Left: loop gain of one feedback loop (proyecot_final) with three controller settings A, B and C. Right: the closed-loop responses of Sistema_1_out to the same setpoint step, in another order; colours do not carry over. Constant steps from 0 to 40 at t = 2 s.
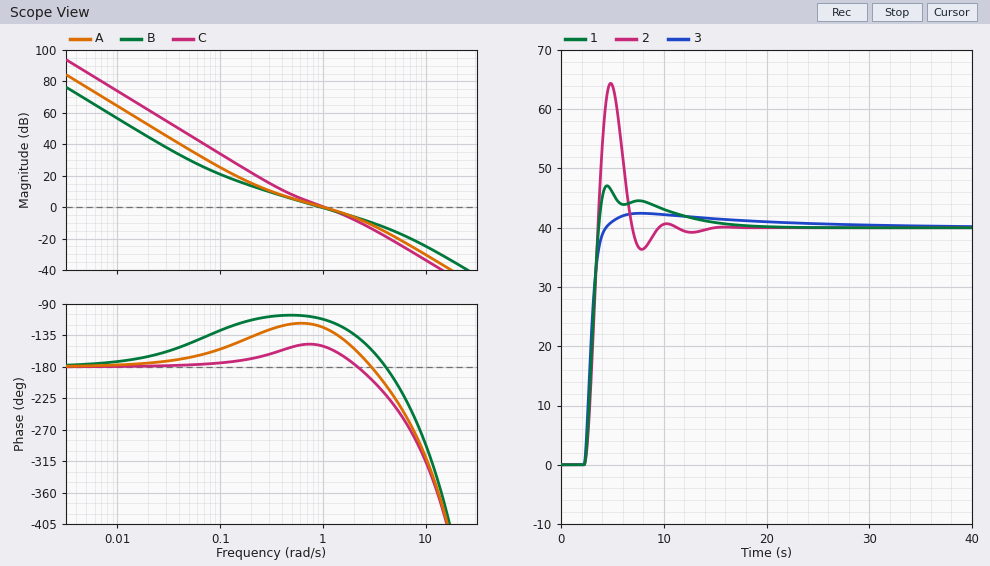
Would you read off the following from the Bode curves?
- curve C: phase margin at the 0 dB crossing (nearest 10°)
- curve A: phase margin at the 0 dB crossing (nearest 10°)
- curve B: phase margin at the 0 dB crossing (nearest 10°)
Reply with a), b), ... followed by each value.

a) 30°
b) 60°
c) 70°
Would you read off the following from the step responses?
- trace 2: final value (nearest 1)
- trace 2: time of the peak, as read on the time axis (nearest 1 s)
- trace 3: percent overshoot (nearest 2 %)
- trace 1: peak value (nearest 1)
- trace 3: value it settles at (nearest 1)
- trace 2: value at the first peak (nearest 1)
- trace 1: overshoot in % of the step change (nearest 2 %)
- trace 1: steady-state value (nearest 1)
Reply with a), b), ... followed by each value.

a) 40
b) 5 s
c) 6 %
d) 47
e) 40
f) 64
g) 18 %
h) 40
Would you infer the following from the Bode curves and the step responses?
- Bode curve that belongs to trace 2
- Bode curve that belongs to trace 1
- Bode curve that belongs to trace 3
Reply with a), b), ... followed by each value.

a) C
b) A
c) B
